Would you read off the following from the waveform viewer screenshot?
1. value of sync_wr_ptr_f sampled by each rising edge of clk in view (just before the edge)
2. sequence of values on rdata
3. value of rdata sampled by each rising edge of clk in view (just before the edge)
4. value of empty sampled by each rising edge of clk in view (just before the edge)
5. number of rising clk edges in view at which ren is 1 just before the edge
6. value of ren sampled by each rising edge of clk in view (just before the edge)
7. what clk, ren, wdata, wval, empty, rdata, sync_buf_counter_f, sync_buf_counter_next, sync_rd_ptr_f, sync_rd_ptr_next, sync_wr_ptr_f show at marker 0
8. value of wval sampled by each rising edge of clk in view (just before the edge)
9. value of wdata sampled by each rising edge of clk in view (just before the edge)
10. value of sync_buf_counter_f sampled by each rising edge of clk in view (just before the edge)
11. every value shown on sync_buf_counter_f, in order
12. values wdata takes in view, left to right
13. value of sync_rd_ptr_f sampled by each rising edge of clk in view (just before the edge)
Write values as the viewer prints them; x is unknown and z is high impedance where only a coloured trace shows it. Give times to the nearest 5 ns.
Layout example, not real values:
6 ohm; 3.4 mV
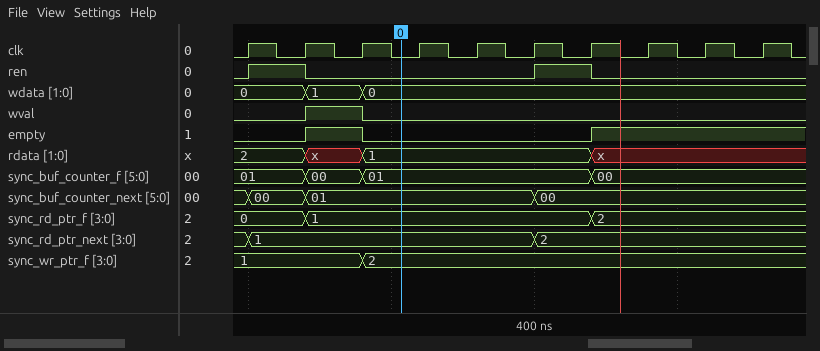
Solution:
1, 1, 1, 2, 2, 2, 2, 2, 2, 2; 2, x, 1, x; 2, 2, x, 1, 1, 1, 1, x, x, x; 0 0 1 0 0 0 0 1 1 1; 2; 0 1 0 0 0 0 1 0 0 0; clk=0, ren=0, wdata=0, wval=0, empty=0, rdata=1, sync_buf_counter_f=01, sync_buf_counter_next=01, sync_rd_ptr_f=1, sync_rd_ptr_next=1, sync_wr_ptr_f=2; 0 0 1 0 0 0 0 0 0 0; 0, 0, 1, 0, 0, 0, 0, 0, 0, 0; 01, 01, 00, 01, 01, 01, 01, 00, 00, 00; 01, 00, 01, 00; 0, 1, 0; 0, 0, 1, 1, 1, 1, 1, 2, 2, 2
